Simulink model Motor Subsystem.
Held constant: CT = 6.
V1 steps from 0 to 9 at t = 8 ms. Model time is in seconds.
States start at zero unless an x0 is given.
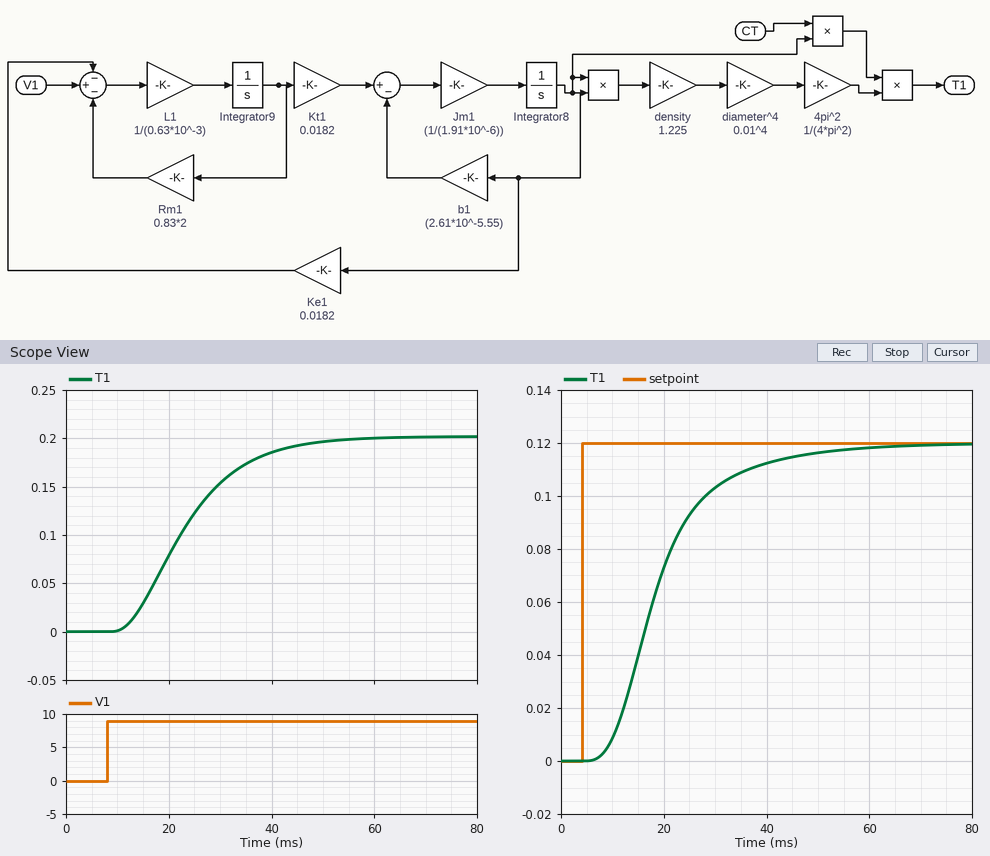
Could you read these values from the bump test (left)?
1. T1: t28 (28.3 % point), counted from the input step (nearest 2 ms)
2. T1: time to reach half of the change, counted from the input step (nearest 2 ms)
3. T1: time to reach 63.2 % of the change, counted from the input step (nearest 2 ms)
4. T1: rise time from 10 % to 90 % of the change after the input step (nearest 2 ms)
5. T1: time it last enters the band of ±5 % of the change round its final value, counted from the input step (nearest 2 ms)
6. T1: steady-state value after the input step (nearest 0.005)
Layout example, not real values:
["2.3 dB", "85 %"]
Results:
["10 ms", "14 ms", "18 ms", "24 ms", "36 ms", "0.200"]
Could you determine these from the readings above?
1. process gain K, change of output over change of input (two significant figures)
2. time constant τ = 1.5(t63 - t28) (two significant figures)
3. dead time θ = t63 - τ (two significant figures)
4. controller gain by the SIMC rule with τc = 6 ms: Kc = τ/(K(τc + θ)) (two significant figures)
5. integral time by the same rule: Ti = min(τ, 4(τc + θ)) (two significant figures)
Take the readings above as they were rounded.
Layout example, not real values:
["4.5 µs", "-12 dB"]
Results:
["0.022", "12 ms", "6.0 ms", "45", "12 ms"]
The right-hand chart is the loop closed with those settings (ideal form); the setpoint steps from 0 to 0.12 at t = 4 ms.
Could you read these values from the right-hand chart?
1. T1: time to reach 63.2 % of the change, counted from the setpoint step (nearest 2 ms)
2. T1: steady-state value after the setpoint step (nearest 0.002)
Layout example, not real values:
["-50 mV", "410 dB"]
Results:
["16 ms", "0.120"]
